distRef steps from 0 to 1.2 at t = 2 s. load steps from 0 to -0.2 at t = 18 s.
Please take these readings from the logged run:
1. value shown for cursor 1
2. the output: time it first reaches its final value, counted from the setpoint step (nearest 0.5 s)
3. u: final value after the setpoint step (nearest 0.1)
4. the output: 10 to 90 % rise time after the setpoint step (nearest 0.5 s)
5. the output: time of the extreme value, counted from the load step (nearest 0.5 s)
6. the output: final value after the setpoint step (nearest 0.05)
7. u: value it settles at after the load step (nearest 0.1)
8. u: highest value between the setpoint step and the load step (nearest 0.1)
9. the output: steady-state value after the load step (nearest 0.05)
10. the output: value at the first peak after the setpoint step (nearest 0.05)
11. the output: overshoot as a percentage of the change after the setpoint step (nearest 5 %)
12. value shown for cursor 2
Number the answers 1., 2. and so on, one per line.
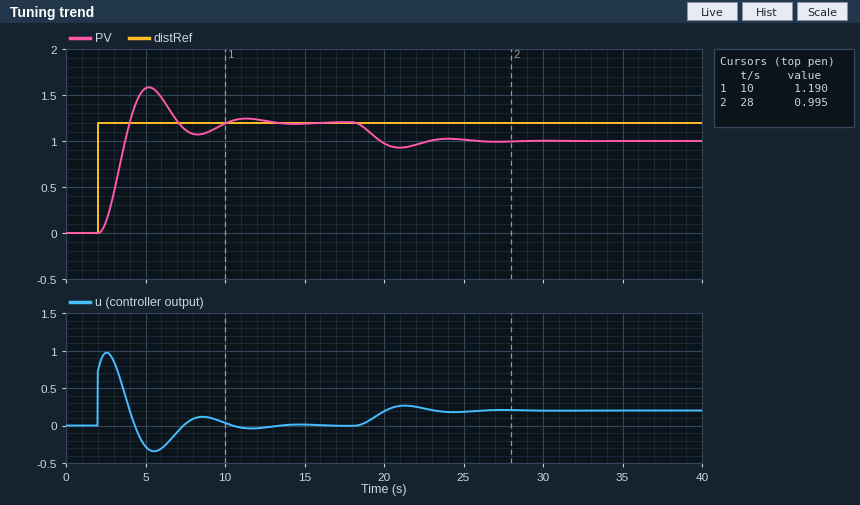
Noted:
1. 1.190
2. 2.0 s
3. 0.0
4. 1.5 s
5. 3.0 s
6. 1.20
7. 0.2
8. 1.0
9. 1.00
10. 1.60
11. 30 %
12. 0.995
